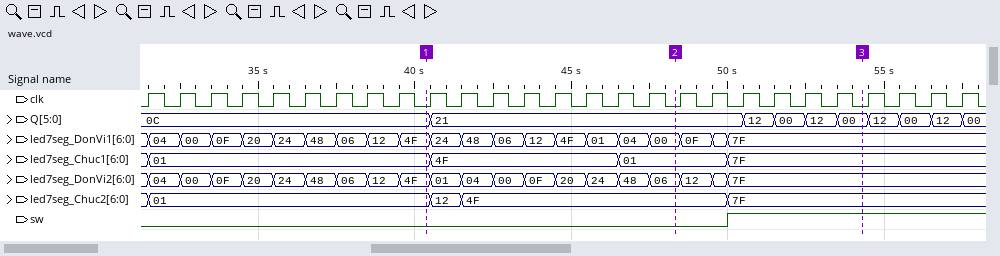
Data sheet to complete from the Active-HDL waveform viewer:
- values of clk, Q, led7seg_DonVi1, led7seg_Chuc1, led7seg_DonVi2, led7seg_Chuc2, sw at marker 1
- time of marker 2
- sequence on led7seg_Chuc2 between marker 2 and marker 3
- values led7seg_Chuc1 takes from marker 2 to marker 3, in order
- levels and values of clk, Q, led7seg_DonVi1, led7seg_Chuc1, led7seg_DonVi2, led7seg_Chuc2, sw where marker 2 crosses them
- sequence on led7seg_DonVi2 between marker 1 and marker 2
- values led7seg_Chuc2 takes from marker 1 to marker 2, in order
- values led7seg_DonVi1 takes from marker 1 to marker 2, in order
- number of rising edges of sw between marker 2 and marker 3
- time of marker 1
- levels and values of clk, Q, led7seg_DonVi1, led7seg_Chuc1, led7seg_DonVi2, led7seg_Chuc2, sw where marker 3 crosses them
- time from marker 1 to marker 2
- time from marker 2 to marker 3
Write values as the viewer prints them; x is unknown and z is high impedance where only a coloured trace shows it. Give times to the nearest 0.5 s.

clk=0, Q=0C, led7seg_DonVi1=4F, led7seg_Chuc1=01, led7seg_DonVi2=4F, led7seg_Chuc2=01, sw=0
48.5 s
4F, 7F
01, 7F
clk=0, Q=21, led7seg_DonVi1=00, led7seg_Chuc1=01, led7seg_DonVi2=06, led7seg_Chuc2=4F, sw=0
4F, 01, 04, 00, 0F, 20, 24, 48, 06
01, 12, 4F
4F, 24, 48, 06, 12, 4F, 01, 04, 00
1
40.5 s
clk=0, Q=00, led7seg_DonVi1=7F, led7seg_Chuc1=7F, led7seg_DonVi2=7F, led7seg_Chuc2=7F, sw=1
8 s
6 s
